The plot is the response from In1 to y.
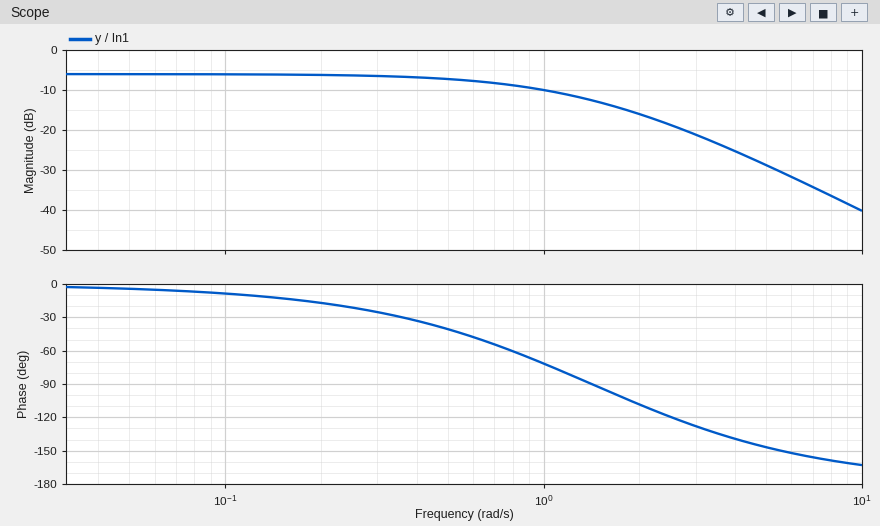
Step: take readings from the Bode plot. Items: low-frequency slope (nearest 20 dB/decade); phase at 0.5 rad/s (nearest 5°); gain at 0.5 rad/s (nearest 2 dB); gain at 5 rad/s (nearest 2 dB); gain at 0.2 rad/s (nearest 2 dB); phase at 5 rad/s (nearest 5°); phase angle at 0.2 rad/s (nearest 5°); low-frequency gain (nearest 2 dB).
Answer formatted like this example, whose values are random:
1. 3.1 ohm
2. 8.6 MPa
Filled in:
1. 0 dB/decade
2. -40°
3. -8 dB
4. -28 dB
5. -6 dB
6. -145°
7. -15°
8. -6 dB
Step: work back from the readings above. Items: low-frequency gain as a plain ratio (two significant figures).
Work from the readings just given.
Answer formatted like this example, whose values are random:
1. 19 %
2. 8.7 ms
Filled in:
1. 0.50
